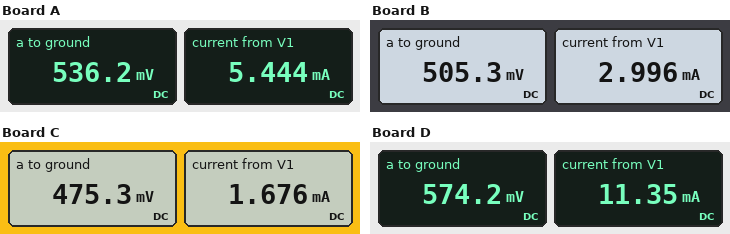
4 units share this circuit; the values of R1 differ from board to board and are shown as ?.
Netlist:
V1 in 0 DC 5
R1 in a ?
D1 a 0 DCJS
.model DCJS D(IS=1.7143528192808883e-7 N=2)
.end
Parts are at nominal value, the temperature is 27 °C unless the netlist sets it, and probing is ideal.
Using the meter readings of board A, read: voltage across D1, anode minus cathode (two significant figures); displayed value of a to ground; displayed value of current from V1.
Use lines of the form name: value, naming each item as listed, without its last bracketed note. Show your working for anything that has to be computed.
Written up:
voltage across D1, anode minus cathode: 536.2 mV = 540 mV
displayed value of a to ground: 536.2 mV
displayed value of current from V1: 5.444 mA
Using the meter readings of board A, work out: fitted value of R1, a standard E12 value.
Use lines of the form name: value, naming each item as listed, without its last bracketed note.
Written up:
fitted value of R1, a standard E12 value: 820 Ω
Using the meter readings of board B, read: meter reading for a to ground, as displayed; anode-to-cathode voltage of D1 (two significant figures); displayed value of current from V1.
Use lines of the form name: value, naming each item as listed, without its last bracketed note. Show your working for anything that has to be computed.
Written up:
meter reading for a to ground, as displayed: 505.3 mV
anode-to-cathode voltage of D1: 505.3 mV = 510 mV
displayed value of current from V1: 2.996 mA
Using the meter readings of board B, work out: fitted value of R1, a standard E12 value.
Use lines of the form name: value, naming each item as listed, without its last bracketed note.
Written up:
fitted value of R1, a standard E12 value: 1.5 kΩ
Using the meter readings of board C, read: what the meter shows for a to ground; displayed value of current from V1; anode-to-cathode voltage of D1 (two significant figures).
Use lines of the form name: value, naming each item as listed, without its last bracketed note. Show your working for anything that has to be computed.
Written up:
what the meter shows for a to ground: 475.3 mV
displayed value of current from V1: 1.676 mA
anode-to-cathode voltage of D1: 475.3 mV = 480 mV
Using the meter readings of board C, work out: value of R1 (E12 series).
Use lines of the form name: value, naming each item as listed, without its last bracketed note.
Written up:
value of R1: 2.7 kΩ
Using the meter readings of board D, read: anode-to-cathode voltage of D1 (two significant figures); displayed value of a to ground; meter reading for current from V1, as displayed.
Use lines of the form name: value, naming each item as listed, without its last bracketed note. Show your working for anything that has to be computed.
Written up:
anode-to-cathode voltage of D1: 574.2 mV = 570 mV
displayed value of a to ground: 574.2 mV
meter reading for current from V1, as displayed: 11.35 mA
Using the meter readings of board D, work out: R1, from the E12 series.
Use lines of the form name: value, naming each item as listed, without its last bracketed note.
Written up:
R1, from the E12 series: 390 Ω
